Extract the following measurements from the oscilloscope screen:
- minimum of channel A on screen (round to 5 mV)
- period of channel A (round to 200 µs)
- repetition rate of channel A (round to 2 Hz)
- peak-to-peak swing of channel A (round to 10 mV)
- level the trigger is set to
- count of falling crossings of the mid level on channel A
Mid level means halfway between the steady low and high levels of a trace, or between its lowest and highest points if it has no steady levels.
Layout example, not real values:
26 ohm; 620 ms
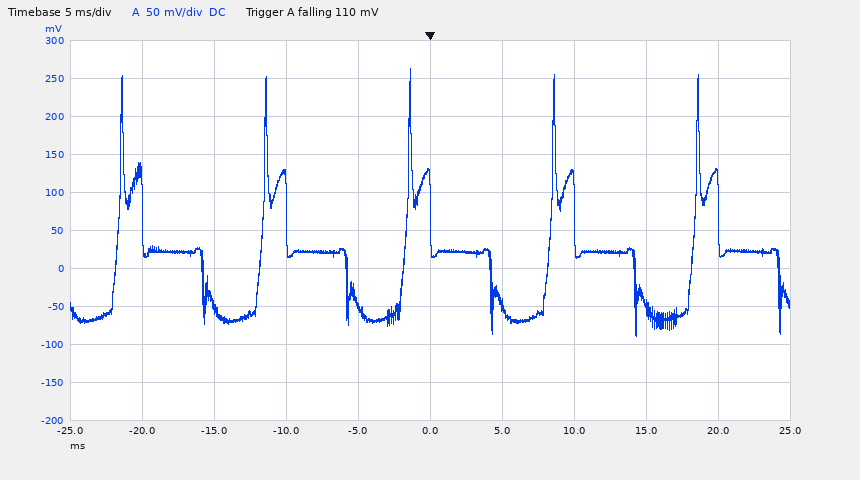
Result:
-90 mV; 10.0 ms; 100 Hz; 350 mV; 110 mV; 5
